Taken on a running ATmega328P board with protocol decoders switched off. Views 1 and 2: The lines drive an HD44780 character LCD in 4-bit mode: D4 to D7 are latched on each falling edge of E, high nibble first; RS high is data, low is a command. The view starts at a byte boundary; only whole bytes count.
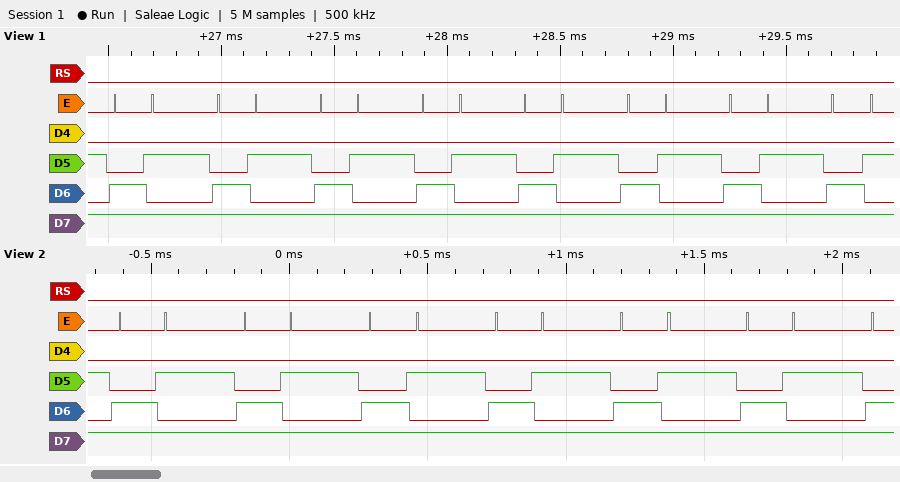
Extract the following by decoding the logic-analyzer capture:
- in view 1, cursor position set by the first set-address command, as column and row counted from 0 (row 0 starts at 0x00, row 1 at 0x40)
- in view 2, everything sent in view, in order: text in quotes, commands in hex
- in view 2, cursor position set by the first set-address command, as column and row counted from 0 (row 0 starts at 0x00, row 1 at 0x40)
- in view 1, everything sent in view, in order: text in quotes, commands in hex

column 10, row 1
0xCA 0xCA 0xCA 0xCA 0xCA 0xCA
column 10, row 1
0xCA 0xCA 0xCA 0xCA 0xCA 0xCA 0xCA 0xCA
